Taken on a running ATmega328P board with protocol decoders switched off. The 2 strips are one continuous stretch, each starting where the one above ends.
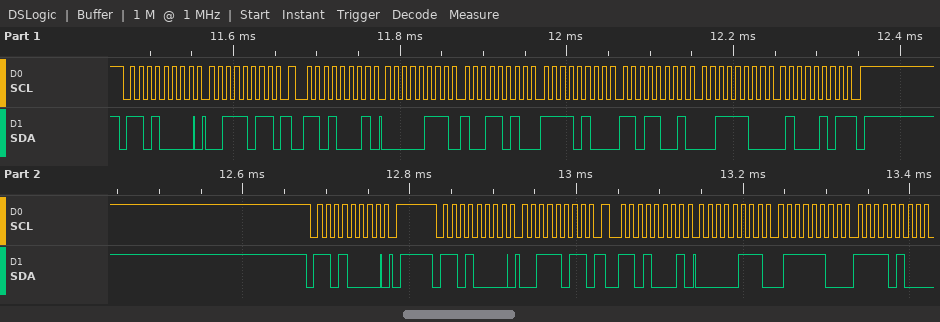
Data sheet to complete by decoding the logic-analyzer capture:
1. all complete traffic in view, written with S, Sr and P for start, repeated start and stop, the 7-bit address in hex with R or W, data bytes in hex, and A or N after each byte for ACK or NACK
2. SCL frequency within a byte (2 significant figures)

S 68W A 3B A Sr 68R A 07 A 9A A F4 A D9 A 3C A 45 N P S 68W A P S 68W A 3B A Sr 68R A 07 A 7C A F4 A
100 kHz
